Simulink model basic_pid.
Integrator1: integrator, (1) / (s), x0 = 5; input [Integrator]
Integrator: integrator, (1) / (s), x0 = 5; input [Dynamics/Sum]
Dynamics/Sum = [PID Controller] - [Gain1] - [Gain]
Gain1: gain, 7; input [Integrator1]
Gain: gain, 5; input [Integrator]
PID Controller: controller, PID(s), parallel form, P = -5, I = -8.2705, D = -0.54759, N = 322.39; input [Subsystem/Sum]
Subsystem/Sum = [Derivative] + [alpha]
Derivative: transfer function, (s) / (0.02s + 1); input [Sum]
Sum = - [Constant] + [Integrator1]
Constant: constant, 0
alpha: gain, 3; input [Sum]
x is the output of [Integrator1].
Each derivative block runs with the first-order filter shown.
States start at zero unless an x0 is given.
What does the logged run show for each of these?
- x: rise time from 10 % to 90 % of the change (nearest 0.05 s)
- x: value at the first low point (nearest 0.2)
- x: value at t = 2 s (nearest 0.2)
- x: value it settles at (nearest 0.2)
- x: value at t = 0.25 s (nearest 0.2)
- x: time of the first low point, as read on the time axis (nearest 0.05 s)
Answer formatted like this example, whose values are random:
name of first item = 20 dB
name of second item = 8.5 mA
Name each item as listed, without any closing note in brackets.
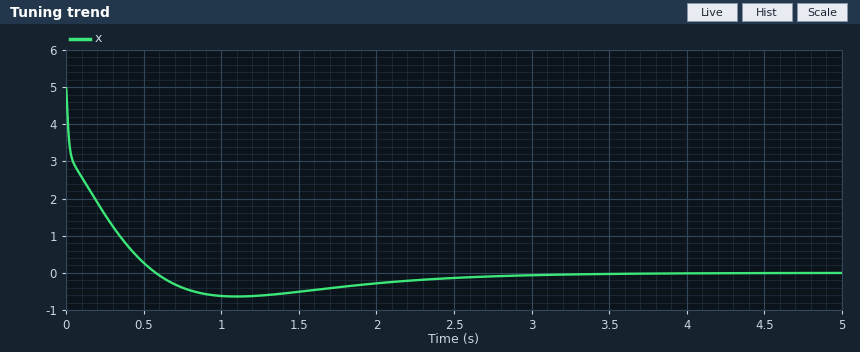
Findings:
x: rise time from 10 % to 90 % of the change = 0.45 s
x: value at the first low point = -0.6
x: value at t = 2 s = -0.2
x: value it settles at = 0.0
x: value at t = 0.25 s = 1.6
x: time of the first low point, as read on the time axis = 1.10 s
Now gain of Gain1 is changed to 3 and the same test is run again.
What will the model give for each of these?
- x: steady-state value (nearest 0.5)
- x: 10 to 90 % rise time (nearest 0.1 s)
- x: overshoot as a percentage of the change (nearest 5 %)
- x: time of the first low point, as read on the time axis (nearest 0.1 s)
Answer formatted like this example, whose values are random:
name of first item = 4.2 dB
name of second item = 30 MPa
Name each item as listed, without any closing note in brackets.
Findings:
x: steady-state value = 0.0
x: 10 to 90 % rise time = 0.5 s
x: overshoot as a percentage of the change = 15 %
x: time of the first low point, as read on the time axis = 1.2 s
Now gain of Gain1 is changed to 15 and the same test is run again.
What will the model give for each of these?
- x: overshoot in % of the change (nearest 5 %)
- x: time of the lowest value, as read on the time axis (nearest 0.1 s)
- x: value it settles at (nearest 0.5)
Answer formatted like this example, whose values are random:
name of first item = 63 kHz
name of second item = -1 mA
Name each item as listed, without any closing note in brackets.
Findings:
x: overshoot in % of the change = 10 %
x: time of the lowest value, as read on the time axis = 0.9 s
x: value it settles at = 0.0
